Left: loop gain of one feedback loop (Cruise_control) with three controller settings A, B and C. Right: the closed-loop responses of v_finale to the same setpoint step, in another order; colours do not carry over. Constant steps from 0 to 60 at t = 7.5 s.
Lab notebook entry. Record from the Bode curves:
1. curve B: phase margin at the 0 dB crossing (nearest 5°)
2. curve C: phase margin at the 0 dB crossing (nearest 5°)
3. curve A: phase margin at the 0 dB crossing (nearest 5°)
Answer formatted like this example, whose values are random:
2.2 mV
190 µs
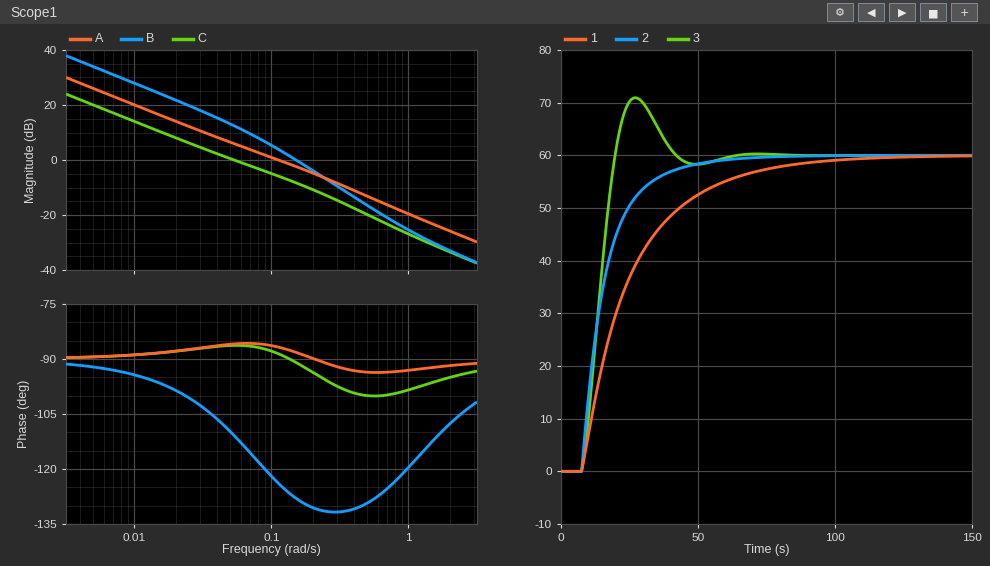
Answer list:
50°
95°
95°
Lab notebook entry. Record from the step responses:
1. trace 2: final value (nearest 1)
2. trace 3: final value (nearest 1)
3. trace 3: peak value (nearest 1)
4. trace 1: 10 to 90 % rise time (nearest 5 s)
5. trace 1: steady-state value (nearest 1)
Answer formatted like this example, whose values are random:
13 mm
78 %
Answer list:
60
60
71
45 s
60
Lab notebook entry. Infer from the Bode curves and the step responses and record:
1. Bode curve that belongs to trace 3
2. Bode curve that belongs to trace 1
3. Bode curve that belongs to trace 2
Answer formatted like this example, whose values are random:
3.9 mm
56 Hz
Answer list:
B
C
A
